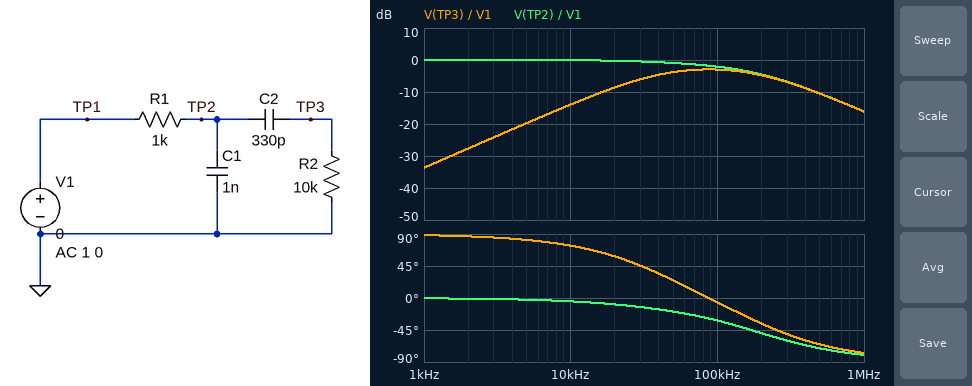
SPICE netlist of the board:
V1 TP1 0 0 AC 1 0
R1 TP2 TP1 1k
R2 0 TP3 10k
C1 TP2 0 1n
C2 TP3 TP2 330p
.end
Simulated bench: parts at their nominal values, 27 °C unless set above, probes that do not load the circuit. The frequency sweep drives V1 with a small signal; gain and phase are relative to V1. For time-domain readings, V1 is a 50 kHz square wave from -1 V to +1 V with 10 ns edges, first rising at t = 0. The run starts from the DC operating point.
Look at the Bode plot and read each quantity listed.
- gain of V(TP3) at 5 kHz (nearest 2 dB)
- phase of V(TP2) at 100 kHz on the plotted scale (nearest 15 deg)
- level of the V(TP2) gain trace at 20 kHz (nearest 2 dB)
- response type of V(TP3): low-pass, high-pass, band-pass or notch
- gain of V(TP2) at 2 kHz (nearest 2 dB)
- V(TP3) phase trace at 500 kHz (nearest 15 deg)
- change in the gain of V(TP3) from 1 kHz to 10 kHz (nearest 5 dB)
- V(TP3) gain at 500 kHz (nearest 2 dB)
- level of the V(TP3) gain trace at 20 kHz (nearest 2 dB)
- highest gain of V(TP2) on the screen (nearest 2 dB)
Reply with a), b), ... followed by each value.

a) -20 dB
b) -30 deg
c) 0 dB
d) band-pass
e) 0 dB
f) -60 deg
g) 20 dB
h) -10 dB
i) -8 dB
j) 0 dB
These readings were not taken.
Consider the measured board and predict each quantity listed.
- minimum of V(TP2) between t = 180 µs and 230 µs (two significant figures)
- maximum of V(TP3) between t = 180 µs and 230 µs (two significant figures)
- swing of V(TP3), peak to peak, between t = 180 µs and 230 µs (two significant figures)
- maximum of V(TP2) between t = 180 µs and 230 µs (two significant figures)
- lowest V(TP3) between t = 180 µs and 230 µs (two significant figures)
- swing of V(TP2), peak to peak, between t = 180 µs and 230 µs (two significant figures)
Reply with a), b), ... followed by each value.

a) -980 mV
b) 1.0 V
c) 2.1 V
d) 980 mV
e) -1.0 V
f) 2.0 V
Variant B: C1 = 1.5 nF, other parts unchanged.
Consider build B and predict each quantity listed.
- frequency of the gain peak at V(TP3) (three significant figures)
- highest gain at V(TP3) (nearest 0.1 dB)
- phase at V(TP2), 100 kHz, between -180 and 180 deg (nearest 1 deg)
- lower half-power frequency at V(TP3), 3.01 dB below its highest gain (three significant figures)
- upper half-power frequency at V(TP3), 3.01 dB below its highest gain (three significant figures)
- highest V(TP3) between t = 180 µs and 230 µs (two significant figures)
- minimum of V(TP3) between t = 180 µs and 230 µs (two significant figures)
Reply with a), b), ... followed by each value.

a) 71.5 kHz
b) -3.8 dB
c) -42 deg
d) 26.7 kHz
e) 192 kHz
f) 890 mV
g) -890 mV
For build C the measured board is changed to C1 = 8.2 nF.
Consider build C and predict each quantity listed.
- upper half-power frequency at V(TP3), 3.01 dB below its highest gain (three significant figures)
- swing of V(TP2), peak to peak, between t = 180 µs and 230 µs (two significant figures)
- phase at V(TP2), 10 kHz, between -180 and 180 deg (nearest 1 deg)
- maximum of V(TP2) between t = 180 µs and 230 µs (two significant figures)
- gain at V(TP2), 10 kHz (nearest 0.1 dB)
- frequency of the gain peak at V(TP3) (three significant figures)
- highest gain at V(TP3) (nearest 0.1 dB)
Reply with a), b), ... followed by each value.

a) 81.1 kHz
b) 1.1 V
c) -28 deg
d) 530 mV
e) -1.1 dB
f) 30.6 kHz
g) -11.1 dB
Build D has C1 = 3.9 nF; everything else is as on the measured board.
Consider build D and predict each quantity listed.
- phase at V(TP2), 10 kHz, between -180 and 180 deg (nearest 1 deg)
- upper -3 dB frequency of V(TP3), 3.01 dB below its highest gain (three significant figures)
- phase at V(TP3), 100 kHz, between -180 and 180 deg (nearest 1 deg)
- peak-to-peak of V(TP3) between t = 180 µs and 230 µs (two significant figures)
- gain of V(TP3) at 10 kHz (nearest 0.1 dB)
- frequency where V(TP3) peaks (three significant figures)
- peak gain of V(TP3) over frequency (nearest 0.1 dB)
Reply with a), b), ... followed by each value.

a) -15 deg
b) 111 kHz
c) -41 deg
d) 1.0 V
e) -14.2 dB
f) 44.4 kHz
g) -7.2 dB
